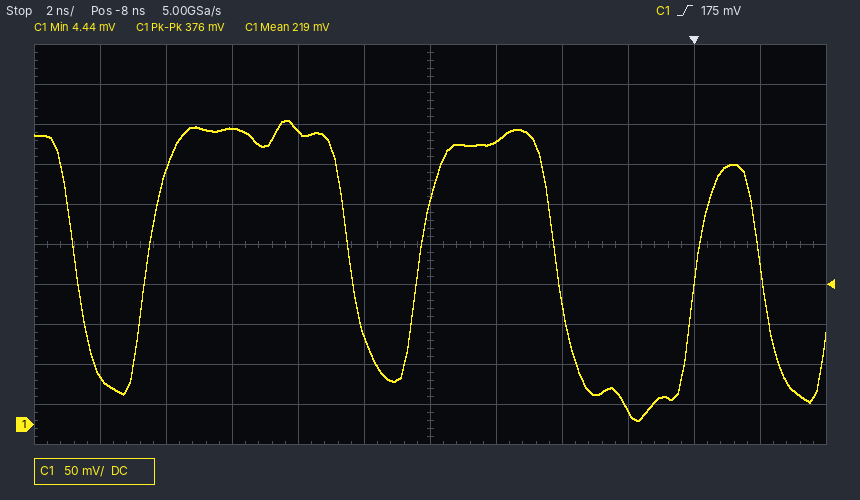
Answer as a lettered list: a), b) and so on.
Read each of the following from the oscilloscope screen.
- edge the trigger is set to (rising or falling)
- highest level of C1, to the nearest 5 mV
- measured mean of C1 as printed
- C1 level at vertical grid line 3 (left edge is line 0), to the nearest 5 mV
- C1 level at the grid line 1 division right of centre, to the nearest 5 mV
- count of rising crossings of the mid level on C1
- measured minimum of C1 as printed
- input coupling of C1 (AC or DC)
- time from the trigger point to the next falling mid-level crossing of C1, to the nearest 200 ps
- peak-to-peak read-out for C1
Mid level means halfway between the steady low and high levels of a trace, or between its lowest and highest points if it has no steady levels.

a) rising
b) 380 mV
c) 219 mV
d) 370 mV
e) 355 mV
f) 3
g) 4.44 mV
h) DC
i) 2.0 ns
j) 376 mV
